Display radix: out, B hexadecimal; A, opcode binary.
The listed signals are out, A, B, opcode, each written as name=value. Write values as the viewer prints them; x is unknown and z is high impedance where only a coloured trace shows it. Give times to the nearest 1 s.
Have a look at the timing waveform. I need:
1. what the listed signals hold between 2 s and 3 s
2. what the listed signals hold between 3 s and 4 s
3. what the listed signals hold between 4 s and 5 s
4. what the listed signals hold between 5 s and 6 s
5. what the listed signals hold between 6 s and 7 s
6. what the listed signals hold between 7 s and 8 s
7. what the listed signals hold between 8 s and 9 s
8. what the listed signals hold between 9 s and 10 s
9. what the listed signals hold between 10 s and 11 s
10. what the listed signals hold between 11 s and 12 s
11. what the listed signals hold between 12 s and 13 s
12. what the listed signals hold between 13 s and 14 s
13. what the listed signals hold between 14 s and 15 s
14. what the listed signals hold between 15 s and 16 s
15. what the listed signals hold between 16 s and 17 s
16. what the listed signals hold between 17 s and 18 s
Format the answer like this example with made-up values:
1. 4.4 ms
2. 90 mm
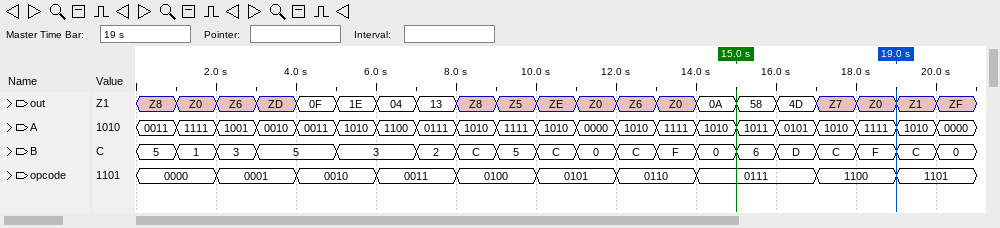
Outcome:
1. out=Z6, A=1001, B=3, opcode=0001
2. out=ZD, A=0010, B=5, opcode=0001
3. out=0F, A=0011, B=5, opcode=0010
4. out=1E, A=1010, B=3, opcode=0010
5. out=04, A=1100, B=3, opcode=0011
6. out=13, A=0111, B=2, opcode=0011
7. out=Z8, A=1010, B=C, opcode=0100
8. out=Z5, A=1111, B=5, opcode=0100
9. out=ZE, A=1010, B=C, opcode=0101
10. out=Z0, A=0000, B=0, opcode=0101
11. out=Z6, A=1010, B=C, opcode=0110
12. out=Z0, A=1111, B=F, opcode=0110
13. out=0A, A=1010, B=0, opcode=0111
14. out=58, A=1011, B=6, opcode=0111
15. out=4D, A=0101, B=D, opcode=0111
16. out=Z7, A=1010, B=C, opcode=1100
